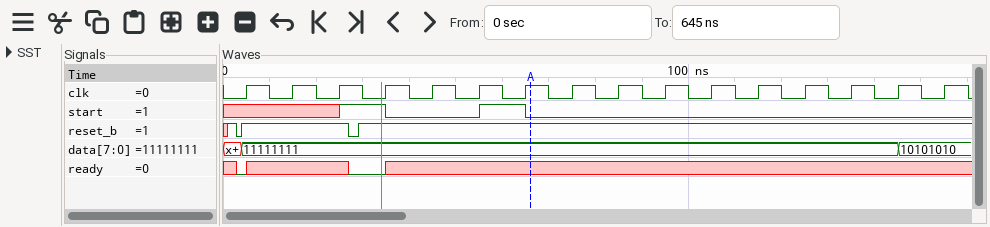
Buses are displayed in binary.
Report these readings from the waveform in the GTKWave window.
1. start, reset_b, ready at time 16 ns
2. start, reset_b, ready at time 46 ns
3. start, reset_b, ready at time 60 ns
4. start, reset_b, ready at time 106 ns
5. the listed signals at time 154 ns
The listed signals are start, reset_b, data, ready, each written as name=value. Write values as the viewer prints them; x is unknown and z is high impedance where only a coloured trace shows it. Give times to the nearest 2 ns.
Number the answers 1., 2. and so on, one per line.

1. start=x, reset_b=1, ready=x
2. start=0, reset_b=1, ready=x
3. start=1, reset_b=1, ready=x
4. start=0, reset_b=1, ready=x
5. start=0, reset_b=1, data=10101010, ready=x
